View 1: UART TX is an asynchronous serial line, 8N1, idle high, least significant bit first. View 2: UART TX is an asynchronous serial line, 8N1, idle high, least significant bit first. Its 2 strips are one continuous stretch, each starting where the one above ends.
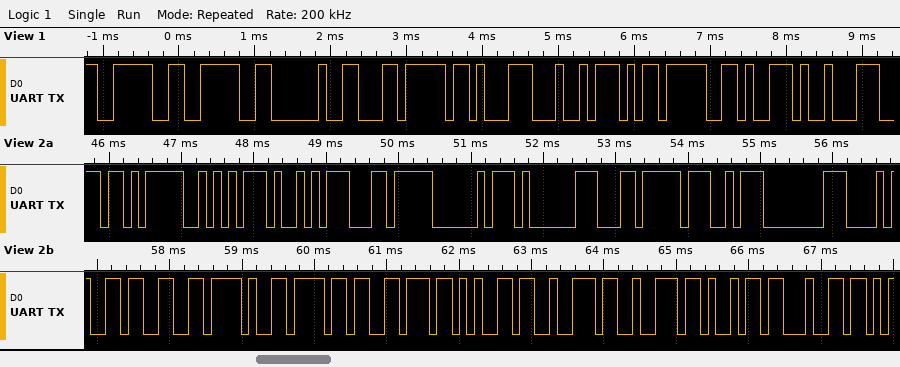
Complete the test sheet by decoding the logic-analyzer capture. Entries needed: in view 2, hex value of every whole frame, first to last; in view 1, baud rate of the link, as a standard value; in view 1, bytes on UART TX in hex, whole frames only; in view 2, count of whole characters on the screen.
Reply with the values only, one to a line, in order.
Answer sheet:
EB AA A9 EC A0 81 EC A7 80 28 33 2F 6F 76 65 72 72 69 64
9600 baud
0x3E 0x3E 0x20 0xEC 0x8B 0xA4 0xED 0x96 0x89
19
